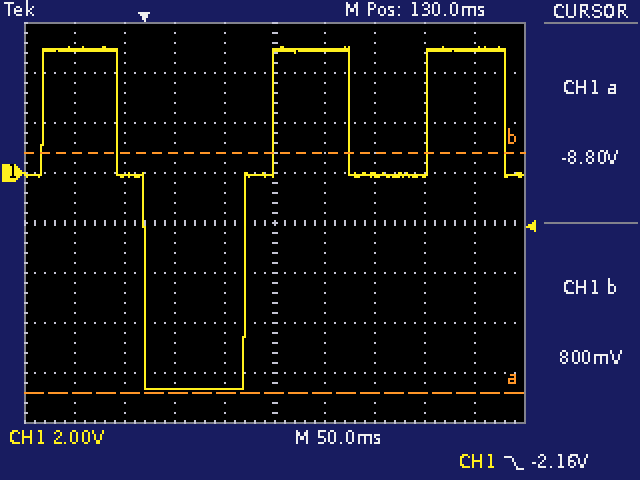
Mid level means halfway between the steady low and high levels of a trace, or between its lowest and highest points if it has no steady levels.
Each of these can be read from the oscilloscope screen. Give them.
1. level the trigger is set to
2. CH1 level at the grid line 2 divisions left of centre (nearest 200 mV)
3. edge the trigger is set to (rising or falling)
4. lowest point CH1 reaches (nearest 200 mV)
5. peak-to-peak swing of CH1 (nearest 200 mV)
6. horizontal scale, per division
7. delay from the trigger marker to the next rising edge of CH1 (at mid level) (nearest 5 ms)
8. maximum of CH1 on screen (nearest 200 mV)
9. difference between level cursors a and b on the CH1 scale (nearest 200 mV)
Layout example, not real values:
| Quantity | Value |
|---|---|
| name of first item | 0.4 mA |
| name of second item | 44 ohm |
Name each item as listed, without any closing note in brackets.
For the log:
| Quantity | Value |
|---|---|
| level the trigger is set to | -2.16 V |
| CH1 level at the grid line 2 divisions left of centre | -8.6 V |
| edge the trigger is set to | falling |
| lowest point CH1 reaches | -8.6 V |
| peak-to-peak swing of CH1 | 13.6 V |
| horizontal scale, per division | 50 ms |
| delay from the trigger marker to the next rising edge of CH1 (at mid level) | 100 ms |
| maximum of CH1 on screen | 5.0 V |
| difference between level cursors a and b on the CH1 scale | 9.6 V |
